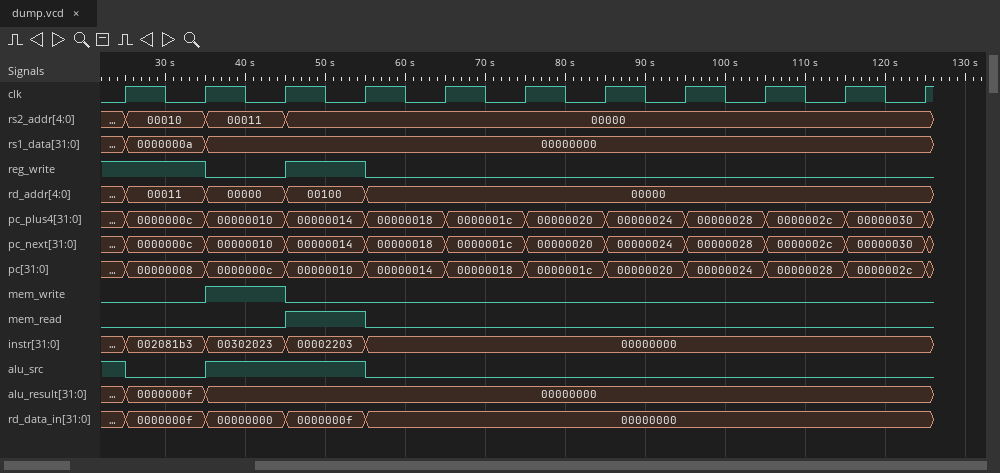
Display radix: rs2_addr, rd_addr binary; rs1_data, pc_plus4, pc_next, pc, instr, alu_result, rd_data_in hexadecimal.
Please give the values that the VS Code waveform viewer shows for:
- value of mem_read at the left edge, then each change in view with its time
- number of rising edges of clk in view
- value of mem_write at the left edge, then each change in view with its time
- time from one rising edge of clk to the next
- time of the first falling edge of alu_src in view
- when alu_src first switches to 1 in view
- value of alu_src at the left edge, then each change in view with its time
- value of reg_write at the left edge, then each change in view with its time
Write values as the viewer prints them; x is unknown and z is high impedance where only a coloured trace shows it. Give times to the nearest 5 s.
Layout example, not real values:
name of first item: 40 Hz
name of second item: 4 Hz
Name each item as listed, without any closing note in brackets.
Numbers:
value of mem_read at the left edge, then each change in view with its time: 0, 1 at 45 s, 0 at 55 s
number of rising edges of clk in view: 11
value of mem_write at the left edge, then each change in view with its time: 0, 1 at 35 s, 0 at 45 s
time from one rising edge of clk to the next: 10 s
time of the first falling edge of alu_src in view: 25 s
when alu_src first switches to 1 in view: 35 s
value of alu_src at the left edge, then each change in view with its time: 1, 0 at 25 s, 1 at 35 s, 0 at 55 s
value of reg_write at the left edge, then each change in view with its time: 1, 0 at 35 s, 1 at 45 s, 0 at 55 s
